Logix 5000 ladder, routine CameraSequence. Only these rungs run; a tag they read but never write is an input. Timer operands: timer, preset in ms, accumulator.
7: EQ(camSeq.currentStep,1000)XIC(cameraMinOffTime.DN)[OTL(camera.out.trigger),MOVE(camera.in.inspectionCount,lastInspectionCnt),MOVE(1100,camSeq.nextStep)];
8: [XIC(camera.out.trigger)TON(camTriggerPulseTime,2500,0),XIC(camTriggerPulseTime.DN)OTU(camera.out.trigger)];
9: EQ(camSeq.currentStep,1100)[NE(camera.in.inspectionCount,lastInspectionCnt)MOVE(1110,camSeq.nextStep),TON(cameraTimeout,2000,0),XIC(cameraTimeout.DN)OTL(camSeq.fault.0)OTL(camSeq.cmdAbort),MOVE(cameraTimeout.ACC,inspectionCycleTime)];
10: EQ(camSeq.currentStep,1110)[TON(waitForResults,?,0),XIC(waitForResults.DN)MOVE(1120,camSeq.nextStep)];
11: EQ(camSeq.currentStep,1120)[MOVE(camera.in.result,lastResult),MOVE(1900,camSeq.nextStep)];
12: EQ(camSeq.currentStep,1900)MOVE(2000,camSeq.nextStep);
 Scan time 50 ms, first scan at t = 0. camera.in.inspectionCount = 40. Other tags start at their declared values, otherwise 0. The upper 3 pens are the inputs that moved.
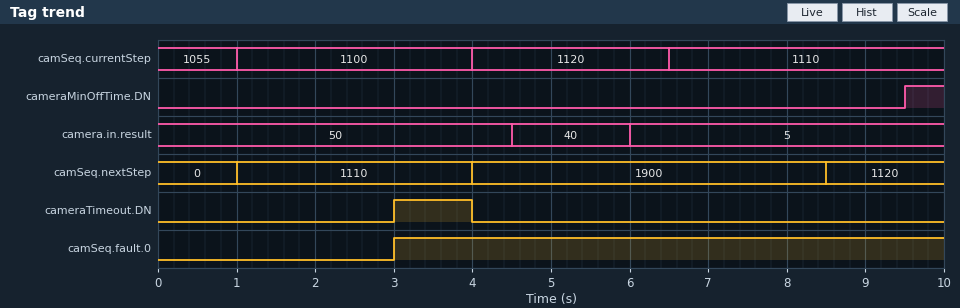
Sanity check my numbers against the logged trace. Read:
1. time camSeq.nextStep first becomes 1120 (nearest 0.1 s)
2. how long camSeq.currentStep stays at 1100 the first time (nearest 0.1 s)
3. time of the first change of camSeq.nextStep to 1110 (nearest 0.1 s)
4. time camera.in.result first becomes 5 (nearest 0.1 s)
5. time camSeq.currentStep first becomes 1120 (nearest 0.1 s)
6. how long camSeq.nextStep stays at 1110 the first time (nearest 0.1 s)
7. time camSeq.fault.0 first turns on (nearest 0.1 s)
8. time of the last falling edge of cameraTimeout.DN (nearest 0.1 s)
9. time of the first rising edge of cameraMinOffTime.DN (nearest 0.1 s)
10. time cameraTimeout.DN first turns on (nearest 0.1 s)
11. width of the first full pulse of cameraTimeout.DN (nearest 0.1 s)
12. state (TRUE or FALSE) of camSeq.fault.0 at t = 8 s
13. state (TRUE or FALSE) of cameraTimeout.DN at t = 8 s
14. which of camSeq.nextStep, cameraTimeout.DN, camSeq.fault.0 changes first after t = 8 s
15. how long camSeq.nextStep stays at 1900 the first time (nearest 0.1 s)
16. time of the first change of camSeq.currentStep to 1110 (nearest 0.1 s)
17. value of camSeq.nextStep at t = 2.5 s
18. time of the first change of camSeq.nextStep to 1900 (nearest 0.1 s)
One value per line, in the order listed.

8.5 s
3.0 s
1.0 s
6.0 s
4.0 s
3.0 s
3.0 s
4.0 s
9.5 s
3.0 s
1.0 s
TRUE
FALSE
camSeq.nextStep
4.5 s
6.5 s
1110
4.0 s
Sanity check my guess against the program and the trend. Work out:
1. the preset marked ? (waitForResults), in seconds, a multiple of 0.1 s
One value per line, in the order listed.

2.0 s
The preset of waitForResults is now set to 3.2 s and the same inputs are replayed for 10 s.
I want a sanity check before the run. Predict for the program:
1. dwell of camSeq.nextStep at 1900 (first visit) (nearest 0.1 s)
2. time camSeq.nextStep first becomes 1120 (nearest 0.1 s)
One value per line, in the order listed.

5.7 s
9.7 s
